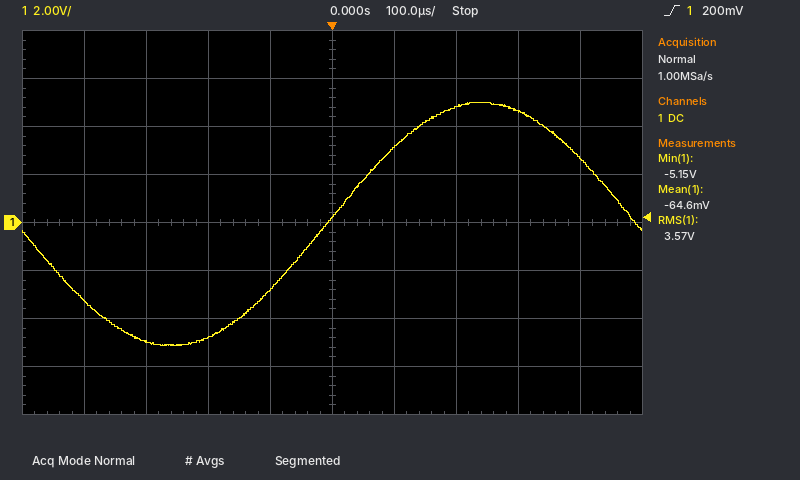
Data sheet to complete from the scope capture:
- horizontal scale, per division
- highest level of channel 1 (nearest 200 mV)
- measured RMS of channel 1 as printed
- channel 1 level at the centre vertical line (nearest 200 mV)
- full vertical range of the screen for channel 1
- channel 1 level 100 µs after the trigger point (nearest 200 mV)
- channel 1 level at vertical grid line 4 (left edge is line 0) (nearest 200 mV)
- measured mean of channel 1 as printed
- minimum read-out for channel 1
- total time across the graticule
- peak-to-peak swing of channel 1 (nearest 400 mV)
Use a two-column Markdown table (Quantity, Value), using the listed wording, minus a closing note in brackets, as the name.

| Quantity | Value |
|---|---|
| horizontal scale, per division | 100 µs |
| highest level of channel 1 | 5.0 V |
| measured RMS of channel 1 as printed | 3.57 V |
| channel 1 level at the centre vertical line | 200 mV |
| full vertical range of the screen for channel 1 | 16 V |
| channel 1 level 100 µs after the trigger point | 3.2 V |
| channel 1 level at vertical grid line 4 (left edge is line 0) | -2.8 V |
| measured mean of channel 1 as printed | -64.6 mV |
| minimum read-out for channel 1 | -5.15 V |
| total time across the graticule | 1 ms |
| peak-to-peak swing of channel 1 | 10.0 V |
